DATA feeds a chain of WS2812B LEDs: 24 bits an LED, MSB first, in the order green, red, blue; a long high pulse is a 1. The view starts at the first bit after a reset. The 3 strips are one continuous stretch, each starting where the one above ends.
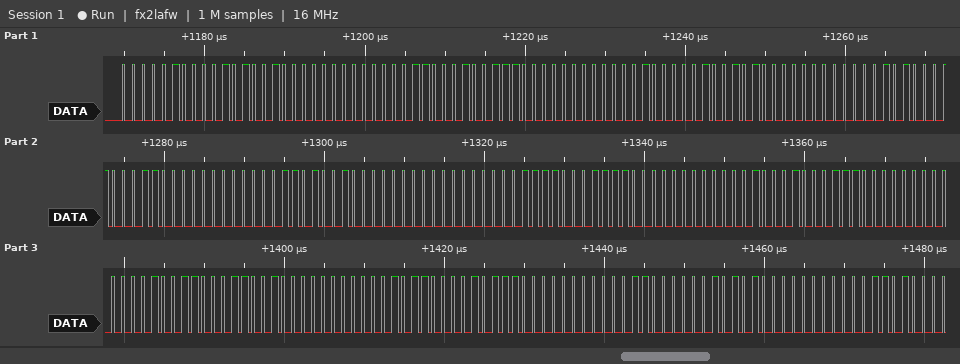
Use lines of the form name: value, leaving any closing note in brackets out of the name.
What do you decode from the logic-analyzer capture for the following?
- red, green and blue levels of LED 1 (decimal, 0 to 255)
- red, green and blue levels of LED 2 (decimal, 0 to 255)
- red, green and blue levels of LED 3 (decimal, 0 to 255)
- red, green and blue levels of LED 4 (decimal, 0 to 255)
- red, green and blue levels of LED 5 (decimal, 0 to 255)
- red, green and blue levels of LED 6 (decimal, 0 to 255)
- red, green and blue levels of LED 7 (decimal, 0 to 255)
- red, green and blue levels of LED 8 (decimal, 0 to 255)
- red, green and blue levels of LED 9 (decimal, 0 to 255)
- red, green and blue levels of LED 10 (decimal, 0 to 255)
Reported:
red, green and blue levels of LED 1: 41, 4, 0
red, green and blue levels of LED 2: 39, 6, 0
red, green and blue levels of LED 3: 37, 8, 0
red, green and blue levels of LED 4: 35, 10, 0
red, green and blue levels of LED 5: 32, 13, 0
red, green and blue levels of LED 6: 30, 15, 0
red, green and blue levels of LED 7: 28, 17, 0
red, green and blue levels of LED 8: 25, 19, 0
red, green and blue levels of LED 9: 23, 22, 0
red, green and blue levels of LED 10: 21, 24, 0
